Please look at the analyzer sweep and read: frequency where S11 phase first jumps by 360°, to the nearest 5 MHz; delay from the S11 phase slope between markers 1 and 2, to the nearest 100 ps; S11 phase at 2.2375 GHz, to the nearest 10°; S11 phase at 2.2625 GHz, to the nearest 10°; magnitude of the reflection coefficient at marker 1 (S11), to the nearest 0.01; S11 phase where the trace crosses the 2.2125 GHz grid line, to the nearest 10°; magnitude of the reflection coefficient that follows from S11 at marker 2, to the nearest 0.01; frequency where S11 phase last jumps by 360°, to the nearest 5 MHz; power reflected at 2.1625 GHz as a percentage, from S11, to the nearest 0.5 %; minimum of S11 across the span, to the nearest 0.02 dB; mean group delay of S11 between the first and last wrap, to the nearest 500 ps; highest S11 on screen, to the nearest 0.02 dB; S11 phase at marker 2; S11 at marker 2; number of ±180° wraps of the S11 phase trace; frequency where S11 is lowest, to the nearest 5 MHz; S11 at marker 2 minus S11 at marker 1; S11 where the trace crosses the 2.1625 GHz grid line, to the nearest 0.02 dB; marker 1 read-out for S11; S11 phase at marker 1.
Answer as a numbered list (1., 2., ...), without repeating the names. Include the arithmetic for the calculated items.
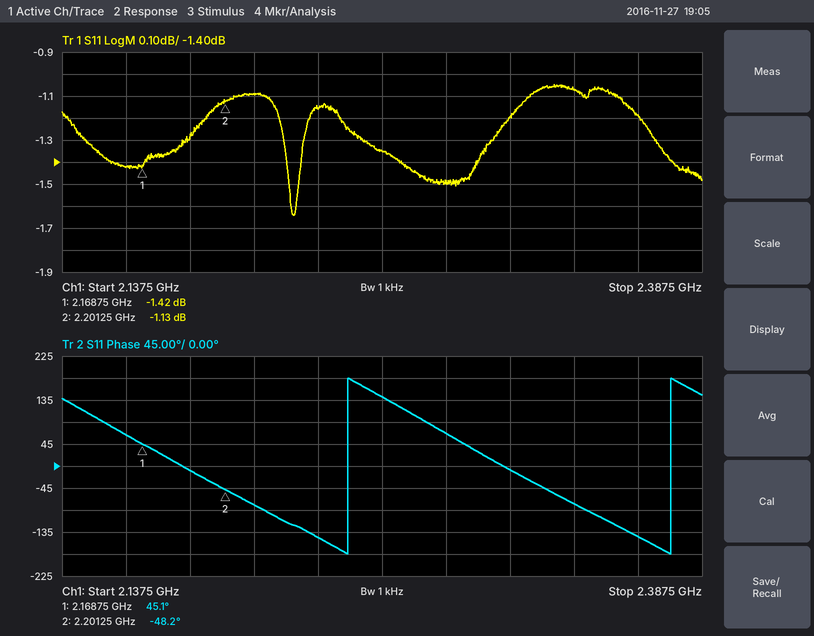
1. 2.250 GHz
2. −(-48.2° − (45.1°))/(360° × 32.5 MHz) ≈ 8.0 ns
3. -150°
4. 140°
5. 10^(-1.42/20) ≈ 0.85
6. -80°
7. 10^(-1.13/20) ≈ 0.88
8. 2.375 GHz
9. 10^(-1.42/10) ≈ 72.1 %, so 72.0 % to the nearest 0.5 %
10. -1.64 dB
11. 1 cycle / (2.375 GHz − 2.250 GHz) ≈ 8.0 ns
12. -1.04 dB
13. -48.2°
14. -1.13 dB
15. 2
16. 2.230 GHz
17. -1.13 − (-1.42) = 0.29 dB
18. -1.42 dB
19. -1.42 dB
20. 45.1°
